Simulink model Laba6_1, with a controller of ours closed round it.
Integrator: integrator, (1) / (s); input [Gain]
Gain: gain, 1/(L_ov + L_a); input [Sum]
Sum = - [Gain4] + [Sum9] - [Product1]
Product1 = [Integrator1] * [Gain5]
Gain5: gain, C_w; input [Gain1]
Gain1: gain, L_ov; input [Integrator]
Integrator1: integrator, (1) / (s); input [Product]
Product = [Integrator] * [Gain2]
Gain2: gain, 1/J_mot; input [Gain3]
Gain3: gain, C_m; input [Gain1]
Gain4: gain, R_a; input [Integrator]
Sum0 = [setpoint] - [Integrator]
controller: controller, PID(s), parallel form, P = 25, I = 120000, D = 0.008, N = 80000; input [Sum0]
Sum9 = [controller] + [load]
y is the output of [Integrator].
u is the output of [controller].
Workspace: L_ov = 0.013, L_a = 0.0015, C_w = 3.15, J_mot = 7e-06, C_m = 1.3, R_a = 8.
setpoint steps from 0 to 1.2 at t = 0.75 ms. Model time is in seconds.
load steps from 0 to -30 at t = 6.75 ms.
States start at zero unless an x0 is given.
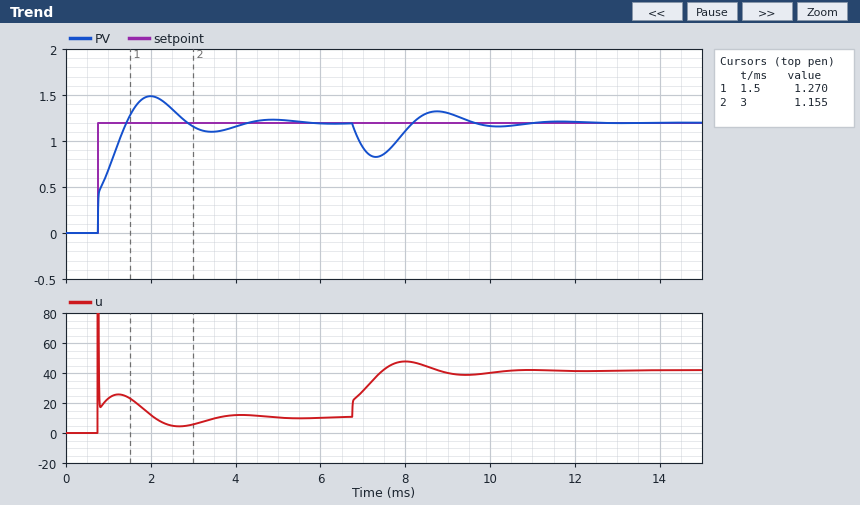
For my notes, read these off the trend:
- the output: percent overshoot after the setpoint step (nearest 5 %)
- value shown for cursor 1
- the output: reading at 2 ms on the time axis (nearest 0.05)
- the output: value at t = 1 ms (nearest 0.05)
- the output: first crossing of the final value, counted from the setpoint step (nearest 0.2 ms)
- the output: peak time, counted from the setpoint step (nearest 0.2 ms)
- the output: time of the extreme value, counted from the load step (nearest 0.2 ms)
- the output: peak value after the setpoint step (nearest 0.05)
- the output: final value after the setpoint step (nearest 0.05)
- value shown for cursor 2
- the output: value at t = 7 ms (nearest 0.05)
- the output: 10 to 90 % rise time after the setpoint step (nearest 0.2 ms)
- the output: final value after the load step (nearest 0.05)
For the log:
25 %
1.270
1.50
0.70
0.6 ms
1.2 ms
0.6 ms
1.50
1.20
1.155
0.95
0.6 ms
1.20
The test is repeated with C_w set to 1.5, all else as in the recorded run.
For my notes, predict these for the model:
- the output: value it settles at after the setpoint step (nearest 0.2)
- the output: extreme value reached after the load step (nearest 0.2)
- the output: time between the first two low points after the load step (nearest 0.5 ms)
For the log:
1.2
0.8
3.0 ms
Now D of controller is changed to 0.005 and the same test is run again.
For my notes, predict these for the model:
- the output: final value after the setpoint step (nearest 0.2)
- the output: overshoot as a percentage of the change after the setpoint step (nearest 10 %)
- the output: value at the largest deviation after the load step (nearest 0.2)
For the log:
1.2
30 %
0.8
